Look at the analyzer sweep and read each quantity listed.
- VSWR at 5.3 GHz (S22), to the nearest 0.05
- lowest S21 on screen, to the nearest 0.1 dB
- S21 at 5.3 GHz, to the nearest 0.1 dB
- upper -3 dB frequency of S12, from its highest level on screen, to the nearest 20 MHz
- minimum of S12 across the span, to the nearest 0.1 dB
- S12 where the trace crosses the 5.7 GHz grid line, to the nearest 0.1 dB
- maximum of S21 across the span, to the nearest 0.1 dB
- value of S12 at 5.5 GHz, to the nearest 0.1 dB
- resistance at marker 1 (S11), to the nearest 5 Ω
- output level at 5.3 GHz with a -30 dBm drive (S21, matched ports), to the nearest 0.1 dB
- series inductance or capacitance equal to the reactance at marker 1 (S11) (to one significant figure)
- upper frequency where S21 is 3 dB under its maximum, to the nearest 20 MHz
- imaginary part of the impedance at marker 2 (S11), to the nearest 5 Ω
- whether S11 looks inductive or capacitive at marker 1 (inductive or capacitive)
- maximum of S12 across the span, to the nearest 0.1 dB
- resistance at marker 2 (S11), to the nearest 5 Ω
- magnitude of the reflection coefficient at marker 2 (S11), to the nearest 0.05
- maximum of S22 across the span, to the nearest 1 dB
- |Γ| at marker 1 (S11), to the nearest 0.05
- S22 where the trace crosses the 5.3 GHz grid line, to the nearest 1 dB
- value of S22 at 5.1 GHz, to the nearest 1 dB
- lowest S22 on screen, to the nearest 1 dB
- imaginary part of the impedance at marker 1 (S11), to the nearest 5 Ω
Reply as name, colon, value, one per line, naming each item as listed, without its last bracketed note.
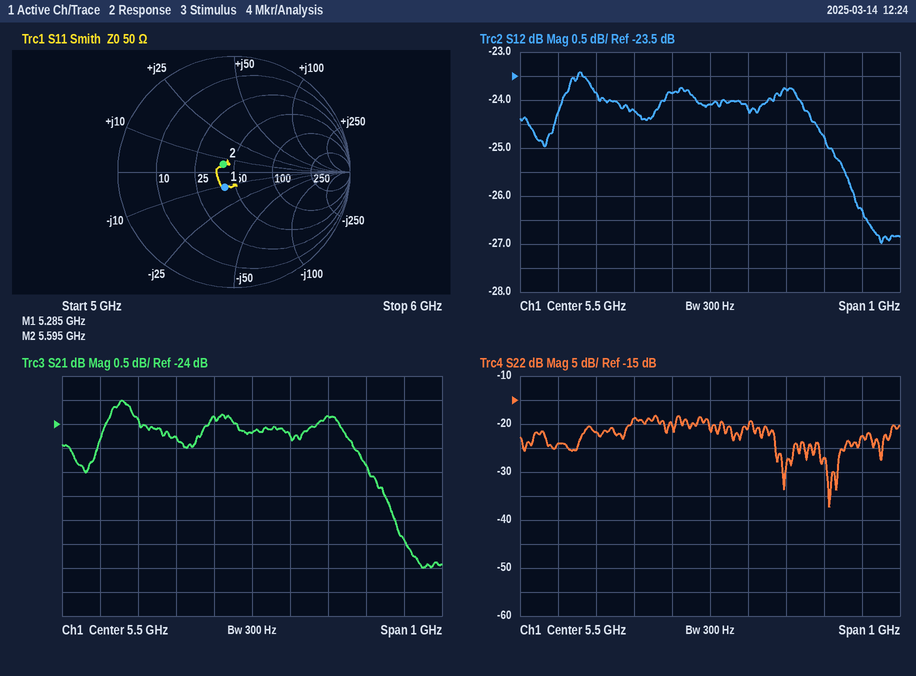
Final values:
VSWR at 5.3 GHz (S22), to the nearest 0.05: 1.25
lowest S21 on screen, to the nearest 0.1 dB: -27.0 dB
S21 at 5.3 GHz, to the nearest 0.1 dB: -24.3 dB
upper -3 dB frequency of S12, from its highest level on screen, to the nearest 20 MHz: 5.90 GHz
minimum of S12 across the span, to the nearest 0.1 dB: -27.0 dB
S12 where the trace crosses the 5.7 GHz grid line, to the nearest 0.1 dB: -23.8 dB
maximum of S21 across the span, to the nearest 0.1 dB: -23.5 dB
value of S12 at 5.5 GHz, to the nearest 0.1 dB: -24.1 dB
resistance at marker 1 (S11), to the nearest 5 Ω: 40 Ω
output level at 5.3 GHz with a -30 dBm drive (S21, matched ports), to the nearest 0.1 dB: -54.3 dBm
series inductance or capacitance equal to the reactance at marker 1 (S11): 3 pF
upper frequency where S21 is 3 dB under its maximum, to the nearest 20 MHz: 5.90 GHz
imaginary part of the impedance at marker 2 (S11), to the nearest 5 Ω: +5 Ω
whether S11 looks inductive or capacitive at marker 1: capacitive
maximum of S12 across the span, to the nearest 0.1 dB: -23.4 dB
resistance at marker 2 (S11), to the nearest 5 Ω: 40 Ω
magnitude of the reflection coefficient at marker 2 (S11), to the nearest 0.05: 0.10
maximum of S22 across the span, to the nearest 1 dB: -18 dB
|Γ| at marker 1 (S11), to the nearest 0.05: 0.15
S22 where the trace crosses the 5.3 GHz grid line, to the nearest 1 dB: -19 dB
value of S22 at 5.1 GHz, to the nearest 1 dB: -24 dB
lowest S22 on screen, to the nearest 1 dB: -37 dB
imaginary part of the impedance at marker 1 (S11), to the nearest 5 Ω: -10 Ω
